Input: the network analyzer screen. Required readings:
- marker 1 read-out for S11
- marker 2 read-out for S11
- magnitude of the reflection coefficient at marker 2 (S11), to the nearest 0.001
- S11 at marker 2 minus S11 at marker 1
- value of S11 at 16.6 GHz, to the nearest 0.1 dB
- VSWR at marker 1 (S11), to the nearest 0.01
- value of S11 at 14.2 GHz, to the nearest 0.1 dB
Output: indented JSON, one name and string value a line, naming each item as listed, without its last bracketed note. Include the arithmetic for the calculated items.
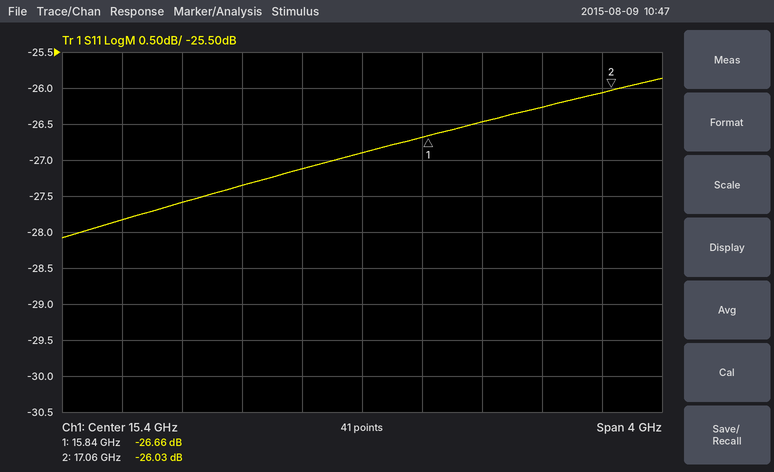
{
  "marker 1 read-out for S11": "-26.66 dB",
  "marker 2 read-out for S11": "-26.03 dB",
  "magnitude of the reflection coefficient at marker 2 (S11), to the nearest 0.001": "10^(-26.03/20) ≈ 0.050",
  "S11 at marker 2 minus S11 at marker 1": "-26.03 − (-26.66) = 0.63 dB",
  "value of S11 at 16.6 GHz, to the nearest 0.1 dB": "-26.3 dB",
  "VSWR at marker 1 (S11), to the nearest 0.01": "(1 + 0.0465)/(1 − 0.0465) ≈ 1.10",
  "value of S11 at 14.2 GHz, to the nearest 0.1 dB": "-27.6 dB"
}
